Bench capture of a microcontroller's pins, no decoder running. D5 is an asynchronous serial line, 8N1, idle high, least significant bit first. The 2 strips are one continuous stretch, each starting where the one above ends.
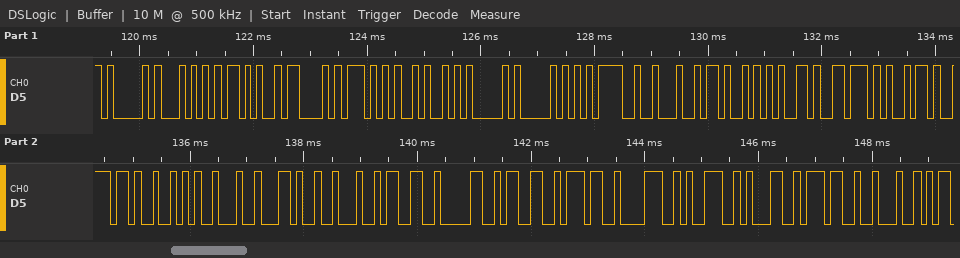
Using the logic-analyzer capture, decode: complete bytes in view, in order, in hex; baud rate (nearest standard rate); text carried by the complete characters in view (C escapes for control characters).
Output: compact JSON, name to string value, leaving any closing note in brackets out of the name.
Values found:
{"complete bytes in view, in order, in hex": "41 54 2B 43 57 4A 41 50 3D 22 4B 65 76 69 6E 52 22 2C 22 33 30 33 37 38 39 31 37 22", "baud rate": "9600 baud", "text carried by the complete characters in view": "\"AT+CWJAP=\\\"KevinR\\\",\\\"30378917\\\"\""}
